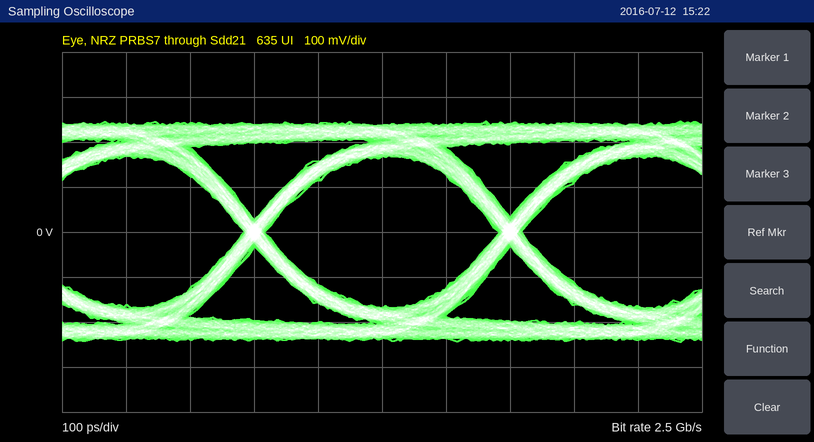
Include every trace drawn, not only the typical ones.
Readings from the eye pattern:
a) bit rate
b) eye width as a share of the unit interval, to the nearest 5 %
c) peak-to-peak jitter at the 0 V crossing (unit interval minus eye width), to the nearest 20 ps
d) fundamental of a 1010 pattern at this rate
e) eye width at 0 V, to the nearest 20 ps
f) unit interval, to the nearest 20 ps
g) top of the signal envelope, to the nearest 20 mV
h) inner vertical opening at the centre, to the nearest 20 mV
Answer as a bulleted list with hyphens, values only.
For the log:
- 2.5 Gb/s
- 90 %
- 40 ps
- 1.25 GHz
- 360 ps
- 400 ps
- 240 mV
- 340 mV
